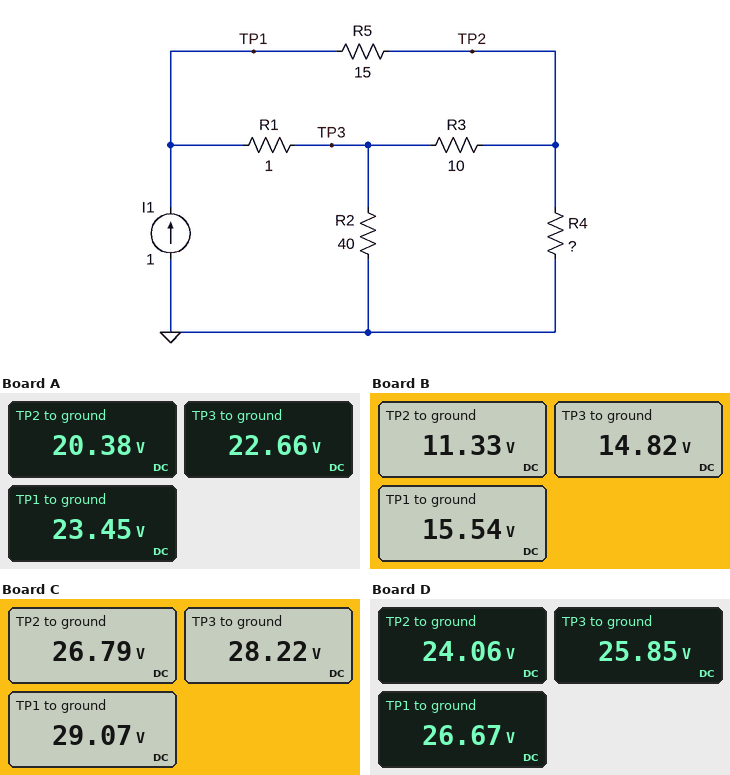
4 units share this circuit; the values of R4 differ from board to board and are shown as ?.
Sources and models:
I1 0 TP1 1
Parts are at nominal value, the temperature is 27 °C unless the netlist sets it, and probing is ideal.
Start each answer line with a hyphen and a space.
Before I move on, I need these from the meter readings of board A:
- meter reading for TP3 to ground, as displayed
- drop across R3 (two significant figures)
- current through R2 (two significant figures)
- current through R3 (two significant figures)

- 22.66 V
- 2.3 V
- 570 mA
- 230 mA
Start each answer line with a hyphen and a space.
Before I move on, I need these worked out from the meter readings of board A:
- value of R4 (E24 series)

- 47 Ω
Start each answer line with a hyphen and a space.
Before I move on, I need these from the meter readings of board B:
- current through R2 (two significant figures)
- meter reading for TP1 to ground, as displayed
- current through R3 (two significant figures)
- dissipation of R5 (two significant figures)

- 370 mA
- 15.54 V
- 350 mA
- 1.2 W
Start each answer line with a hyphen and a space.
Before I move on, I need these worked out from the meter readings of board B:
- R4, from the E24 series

- 18 Ω
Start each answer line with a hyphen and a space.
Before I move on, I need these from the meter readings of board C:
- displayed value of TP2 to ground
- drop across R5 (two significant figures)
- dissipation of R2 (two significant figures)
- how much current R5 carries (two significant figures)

- 26.79 V
- 2.3 V
- 20 W
- 150 mA
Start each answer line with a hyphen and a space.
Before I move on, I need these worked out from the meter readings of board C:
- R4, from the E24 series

- 91 Ω
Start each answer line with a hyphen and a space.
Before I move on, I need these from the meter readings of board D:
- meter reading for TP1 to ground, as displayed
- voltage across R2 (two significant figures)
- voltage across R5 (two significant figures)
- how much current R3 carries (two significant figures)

- 26.67 V
- 26 V
- 2.6 V
- 180 mA
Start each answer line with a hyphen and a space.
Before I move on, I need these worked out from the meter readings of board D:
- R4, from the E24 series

- 68 Ω
